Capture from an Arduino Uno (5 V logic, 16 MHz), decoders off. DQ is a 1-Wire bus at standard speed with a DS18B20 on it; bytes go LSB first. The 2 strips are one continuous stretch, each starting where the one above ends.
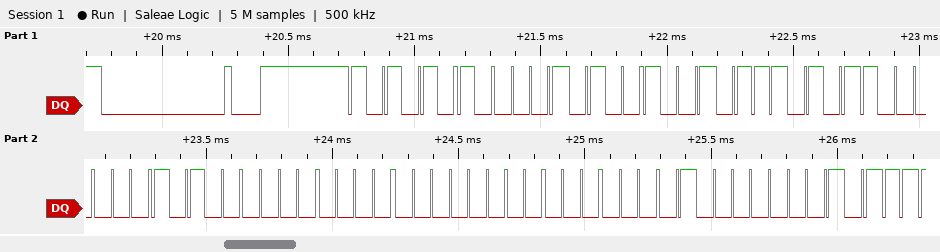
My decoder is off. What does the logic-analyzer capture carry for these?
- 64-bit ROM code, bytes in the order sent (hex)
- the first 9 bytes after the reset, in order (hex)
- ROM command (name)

28 E9 1A 28 00 00 80 80
55 28 E9 1A 28 00 00 80 80
Match ROM
